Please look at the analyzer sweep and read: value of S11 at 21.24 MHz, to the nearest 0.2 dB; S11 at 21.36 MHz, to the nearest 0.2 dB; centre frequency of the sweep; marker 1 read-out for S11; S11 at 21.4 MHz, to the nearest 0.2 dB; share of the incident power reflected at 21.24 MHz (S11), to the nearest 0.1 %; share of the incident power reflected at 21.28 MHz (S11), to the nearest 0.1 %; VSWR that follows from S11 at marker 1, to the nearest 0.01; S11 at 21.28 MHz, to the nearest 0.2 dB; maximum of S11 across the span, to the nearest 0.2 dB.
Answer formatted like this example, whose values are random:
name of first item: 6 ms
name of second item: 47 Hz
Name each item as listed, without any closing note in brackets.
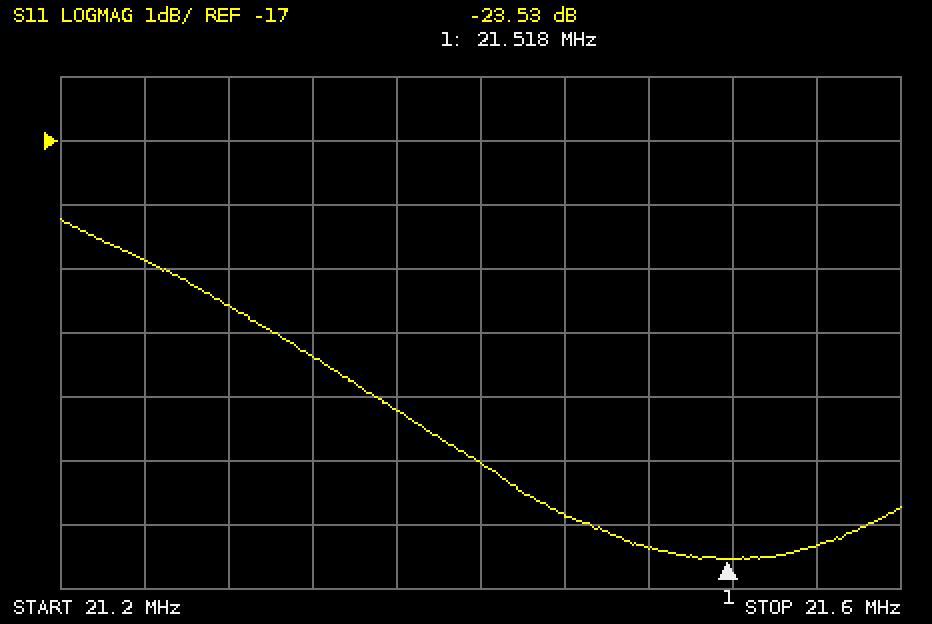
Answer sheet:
value of S11 at 21.24 MHz, to the nearest 0.2 dB: -18.8 dB
S11 at 21.36 MHz, to the nearest 0.2 dB: -21.2 dB
centre frequency of the sweep: 21.4 MHz
marker 1 read-out for S11: -23.53 dB
S11 at 21.4 MHz, to the nearest 0.2 dB: -22.0 dB
share of the incident power reflected at 21.24 MHz (S11), to the nearest 0.1 %: 1.3 %
share of the incident power reflected at 21.28 MHz (S11), to the nearest 0.1 %: 1.1 %
VSWR that follows from S11 at marker 1, to the nearest 0.01: 1.14
S11 at 21.28 MHz, to the nearest 0.2 dB: -19.6 dB
maximum of S11 across the span, to the nearest 0.2 dB: -18.2 dB
